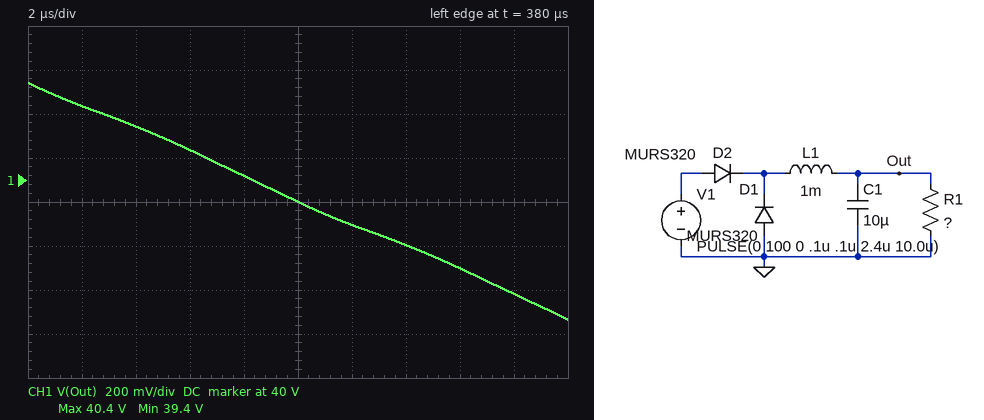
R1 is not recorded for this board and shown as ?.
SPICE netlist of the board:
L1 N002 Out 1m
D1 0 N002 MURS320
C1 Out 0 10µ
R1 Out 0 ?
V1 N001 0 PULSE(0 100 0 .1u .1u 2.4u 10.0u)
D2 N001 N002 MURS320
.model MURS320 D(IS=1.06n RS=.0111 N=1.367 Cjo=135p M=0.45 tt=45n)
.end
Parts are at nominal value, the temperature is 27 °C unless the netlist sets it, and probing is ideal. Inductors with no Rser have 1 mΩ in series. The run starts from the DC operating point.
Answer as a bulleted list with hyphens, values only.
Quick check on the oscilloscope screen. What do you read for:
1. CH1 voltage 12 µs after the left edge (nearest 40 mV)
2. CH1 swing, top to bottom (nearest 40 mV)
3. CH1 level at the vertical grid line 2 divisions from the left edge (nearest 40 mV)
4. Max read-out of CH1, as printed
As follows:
- 39.80 V
- 1.08 V
- 40.24 V
- 40.4 V
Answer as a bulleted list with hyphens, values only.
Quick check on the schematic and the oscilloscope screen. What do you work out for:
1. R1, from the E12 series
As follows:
- 68 Ω
